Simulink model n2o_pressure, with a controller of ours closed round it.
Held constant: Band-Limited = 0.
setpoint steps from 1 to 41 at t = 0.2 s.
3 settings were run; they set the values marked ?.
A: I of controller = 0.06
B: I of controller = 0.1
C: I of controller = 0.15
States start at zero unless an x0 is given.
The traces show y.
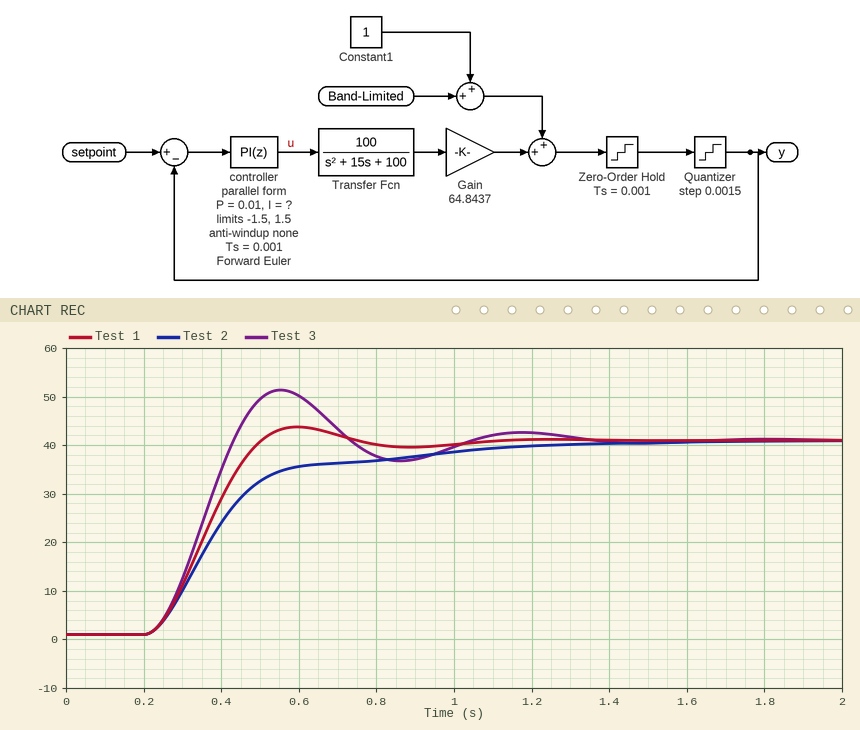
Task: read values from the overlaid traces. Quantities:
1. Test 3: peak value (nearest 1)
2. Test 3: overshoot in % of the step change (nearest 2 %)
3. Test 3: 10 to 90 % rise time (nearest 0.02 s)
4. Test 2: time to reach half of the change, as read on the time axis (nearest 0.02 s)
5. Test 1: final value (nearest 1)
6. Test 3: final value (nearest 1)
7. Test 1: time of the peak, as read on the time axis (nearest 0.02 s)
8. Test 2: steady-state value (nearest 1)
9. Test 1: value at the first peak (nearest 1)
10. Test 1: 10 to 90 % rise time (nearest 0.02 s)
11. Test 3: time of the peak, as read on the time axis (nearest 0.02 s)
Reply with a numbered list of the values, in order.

1. 51
2. 26 %
3. 0.16 s
4. 0.38 s
5. 41
6. 41
7. 0.60 s
8. 41
9. 44
10. 0.20 s
11. 0.56 s
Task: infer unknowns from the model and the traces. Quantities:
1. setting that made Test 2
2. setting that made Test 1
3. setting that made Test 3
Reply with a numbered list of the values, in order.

1. A
2. B
3. C
